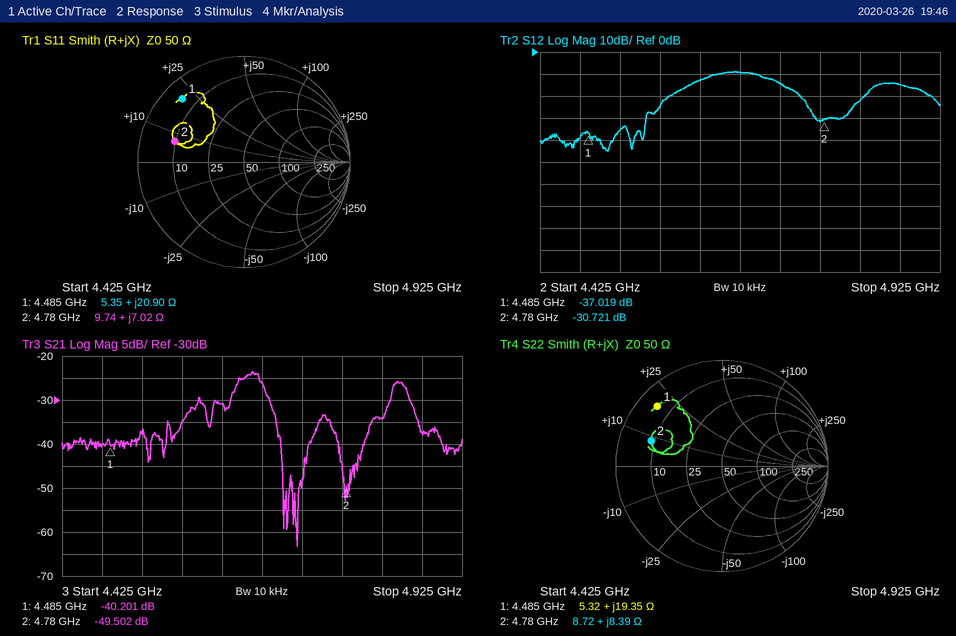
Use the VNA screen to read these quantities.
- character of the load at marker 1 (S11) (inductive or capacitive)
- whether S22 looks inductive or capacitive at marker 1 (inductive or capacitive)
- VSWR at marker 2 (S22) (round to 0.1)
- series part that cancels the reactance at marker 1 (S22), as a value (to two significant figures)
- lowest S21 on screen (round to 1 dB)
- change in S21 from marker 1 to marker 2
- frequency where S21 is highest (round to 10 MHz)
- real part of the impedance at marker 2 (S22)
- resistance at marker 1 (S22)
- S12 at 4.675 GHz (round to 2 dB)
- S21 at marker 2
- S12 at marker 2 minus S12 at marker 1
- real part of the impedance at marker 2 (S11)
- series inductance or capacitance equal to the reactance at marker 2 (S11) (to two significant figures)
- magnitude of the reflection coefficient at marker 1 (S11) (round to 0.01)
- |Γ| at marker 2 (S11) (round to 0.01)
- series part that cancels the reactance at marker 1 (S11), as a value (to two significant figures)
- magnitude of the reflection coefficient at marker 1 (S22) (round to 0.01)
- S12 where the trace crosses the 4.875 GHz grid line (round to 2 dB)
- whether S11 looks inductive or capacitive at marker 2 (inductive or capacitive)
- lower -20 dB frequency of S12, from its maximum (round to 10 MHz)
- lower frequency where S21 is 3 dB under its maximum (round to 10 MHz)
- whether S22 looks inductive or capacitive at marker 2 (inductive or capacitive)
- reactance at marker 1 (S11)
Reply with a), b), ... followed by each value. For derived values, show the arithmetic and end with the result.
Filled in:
a) inductive
b) inductive
c) 5.9
d) C = 1/(2π × 4.485 GHz × 19.35 Ω) ≈ 1.8 pF
e) -63 dB
f) -49.502 − (-40.201) = -9.301 dB
g) 4.66 GHz
h) 8.72 Ω
i) 5.32 Ω
j) -10 dB
k) -49.502 dB
l) -30.721 − (-37.019) = 6.298 dB
m) 9.74 Ω
n) L = 7.02 Ω/(2π × 4.78 GHz) ≈ 234 pH, so 230 pH to two significant figures
o) 0.83
p) 0.68
q) C = 1/(2π × 4.485 GHz × 20.9 Ω) ≈ 1.7 pF
r) 0.83
s) -14 dB
t) inductive
u) 4.56 GHz
v) 4.64 GHz
w) inductive
x) +20.90 Ω
